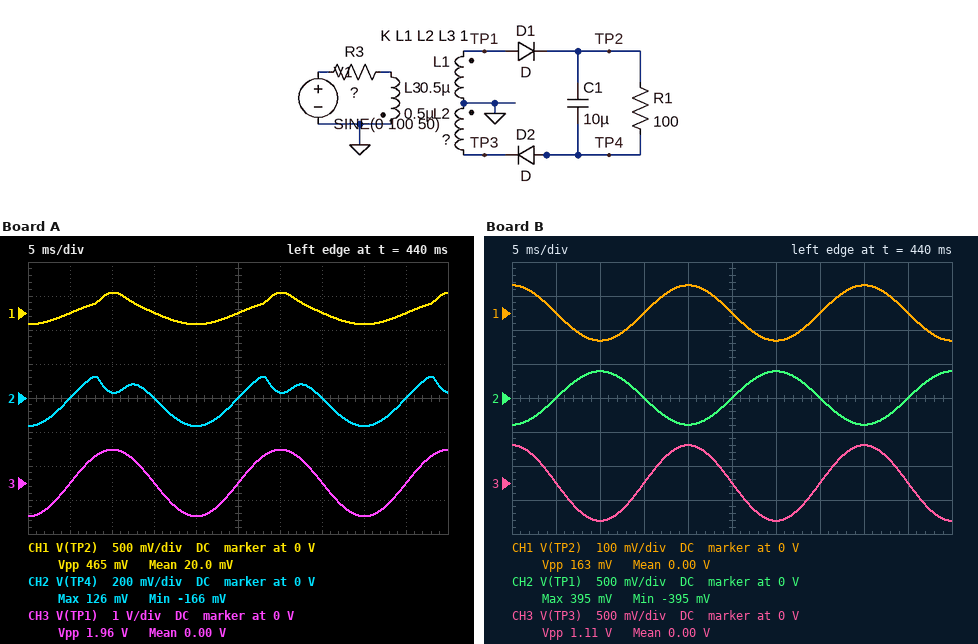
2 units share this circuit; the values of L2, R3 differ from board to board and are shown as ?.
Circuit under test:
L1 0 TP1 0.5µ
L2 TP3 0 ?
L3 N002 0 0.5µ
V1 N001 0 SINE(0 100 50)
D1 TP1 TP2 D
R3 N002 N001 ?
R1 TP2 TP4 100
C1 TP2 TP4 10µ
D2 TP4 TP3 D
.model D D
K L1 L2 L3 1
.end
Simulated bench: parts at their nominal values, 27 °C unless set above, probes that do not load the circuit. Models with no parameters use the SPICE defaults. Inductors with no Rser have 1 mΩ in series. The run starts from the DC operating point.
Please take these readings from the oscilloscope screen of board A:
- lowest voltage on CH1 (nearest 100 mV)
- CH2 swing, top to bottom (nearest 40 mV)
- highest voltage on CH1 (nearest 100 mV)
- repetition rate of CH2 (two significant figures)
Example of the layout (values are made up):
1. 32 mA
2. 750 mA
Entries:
1. -200 mV
2. 280 mV
3. 300 mV
4. 50 Hz
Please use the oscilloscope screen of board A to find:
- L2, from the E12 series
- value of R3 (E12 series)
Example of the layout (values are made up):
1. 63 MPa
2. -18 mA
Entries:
1. 220 nH
2. 0.015 Ω
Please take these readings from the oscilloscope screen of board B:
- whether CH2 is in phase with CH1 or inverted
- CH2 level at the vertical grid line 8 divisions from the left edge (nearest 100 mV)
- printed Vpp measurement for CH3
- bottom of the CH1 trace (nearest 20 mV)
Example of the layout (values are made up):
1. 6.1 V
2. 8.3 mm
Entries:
1. inverted
2. -400 mV
3. 1.11 V
4. -80 mV
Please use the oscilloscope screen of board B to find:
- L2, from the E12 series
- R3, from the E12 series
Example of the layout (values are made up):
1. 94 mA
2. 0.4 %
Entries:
1. 1 µH
2. 0.039 Ω
